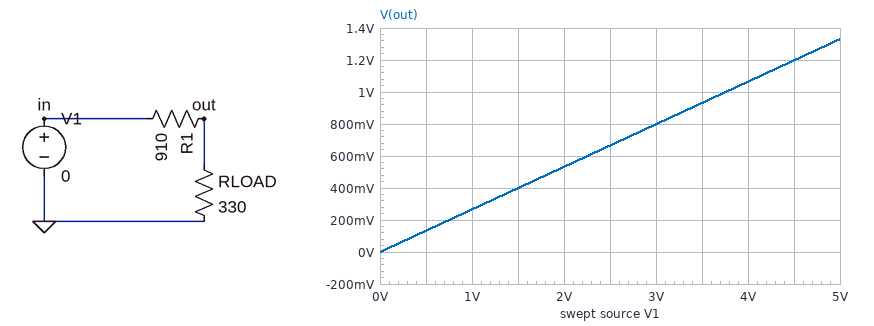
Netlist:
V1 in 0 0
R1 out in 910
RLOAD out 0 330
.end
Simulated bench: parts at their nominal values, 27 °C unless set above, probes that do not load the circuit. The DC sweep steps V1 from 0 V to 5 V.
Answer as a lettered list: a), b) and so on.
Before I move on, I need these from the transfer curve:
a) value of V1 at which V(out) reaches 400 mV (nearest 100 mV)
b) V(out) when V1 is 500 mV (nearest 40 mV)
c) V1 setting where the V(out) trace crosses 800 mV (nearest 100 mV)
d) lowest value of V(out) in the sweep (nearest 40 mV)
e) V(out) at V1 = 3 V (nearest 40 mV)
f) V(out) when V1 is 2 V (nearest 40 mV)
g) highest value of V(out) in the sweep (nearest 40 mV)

a) 1.5 V
b) 120 mV
c) 3.0 V
d) 0 V
e) 800 mV
f) 520 mV
g) 1.32 V
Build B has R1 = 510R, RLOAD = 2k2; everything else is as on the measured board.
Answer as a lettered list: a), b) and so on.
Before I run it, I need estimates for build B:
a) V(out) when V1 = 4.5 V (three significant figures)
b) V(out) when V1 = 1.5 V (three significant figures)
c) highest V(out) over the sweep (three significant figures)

a) 3.65 V
b) 1.22 V
c) 4.06 V
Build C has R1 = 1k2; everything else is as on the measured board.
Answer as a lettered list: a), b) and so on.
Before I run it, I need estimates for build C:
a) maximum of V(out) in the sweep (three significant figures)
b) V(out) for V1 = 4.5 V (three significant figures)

a) 1.08 V
b) 971 mV
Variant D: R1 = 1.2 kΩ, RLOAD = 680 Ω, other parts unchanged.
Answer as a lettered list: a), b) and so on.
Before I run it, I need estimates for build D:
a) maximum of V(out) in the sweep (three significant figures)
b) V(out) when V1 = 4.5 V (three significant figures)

a) 1.81 V
b) 1.63 V
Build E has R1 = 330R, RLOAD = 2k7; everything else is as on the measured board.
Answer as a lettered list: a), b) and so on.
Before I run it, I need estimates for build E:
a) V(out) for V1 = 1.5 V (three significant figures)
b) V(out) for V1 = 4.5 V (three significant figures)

a) 1.34 V
b) 4.01 V
